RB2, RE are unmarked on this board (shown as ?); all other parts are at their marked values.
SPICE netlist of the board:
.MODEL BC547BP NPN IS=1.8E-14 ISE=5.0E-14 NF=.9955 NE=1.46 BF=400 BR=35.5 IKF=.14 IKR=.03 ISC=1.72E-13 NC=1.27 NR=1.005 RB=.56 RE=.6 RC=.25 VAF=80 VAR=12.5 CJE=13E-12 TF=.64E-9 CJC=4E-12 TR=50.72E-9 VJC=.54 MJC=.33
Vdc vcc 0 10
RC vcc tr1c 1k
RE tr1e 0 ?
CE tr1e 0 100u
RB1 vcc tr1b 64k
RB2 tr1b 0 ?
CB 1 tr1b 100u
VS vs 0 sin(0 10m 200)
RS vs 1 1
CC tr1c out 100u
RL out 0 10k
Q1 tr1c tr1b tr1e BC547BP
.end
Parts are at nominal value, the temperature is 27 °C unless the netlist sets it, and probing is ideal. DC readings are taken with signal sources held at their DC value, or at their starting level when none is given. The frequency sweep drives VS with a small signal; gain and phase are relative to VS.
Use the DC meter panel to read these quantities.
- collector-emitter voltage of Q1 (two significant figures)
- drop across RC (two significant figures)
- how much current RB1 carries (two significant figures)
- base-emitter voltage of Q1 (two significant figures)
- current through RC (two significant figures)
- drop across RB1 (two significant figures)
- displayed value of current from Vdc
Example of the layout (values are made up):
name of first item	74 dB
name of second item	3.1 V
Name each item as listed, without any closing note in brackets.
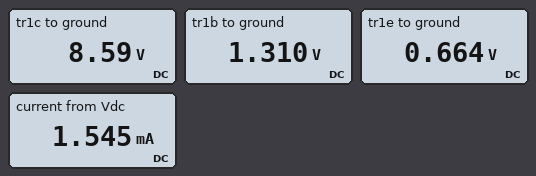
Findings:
collector-emitter voltage of Q1	7.9 V
drop across RC	1.4 V
how much current RB1 carries	140 µA
base-emitter voltage of Q1	650 mV
current through RC	1.4 mA
drop across RB1	8.7 V
displayed value of current from Vdc	1.545 mA
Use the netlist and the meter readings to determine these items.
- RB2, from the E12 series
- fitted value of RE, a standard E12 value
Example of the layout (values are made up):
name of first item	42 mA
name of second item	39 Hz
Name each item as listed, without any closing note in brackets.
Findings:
RB2, from the E12 series	10 kΩ
fitted value of RE, a standard E12 value	470 Ω
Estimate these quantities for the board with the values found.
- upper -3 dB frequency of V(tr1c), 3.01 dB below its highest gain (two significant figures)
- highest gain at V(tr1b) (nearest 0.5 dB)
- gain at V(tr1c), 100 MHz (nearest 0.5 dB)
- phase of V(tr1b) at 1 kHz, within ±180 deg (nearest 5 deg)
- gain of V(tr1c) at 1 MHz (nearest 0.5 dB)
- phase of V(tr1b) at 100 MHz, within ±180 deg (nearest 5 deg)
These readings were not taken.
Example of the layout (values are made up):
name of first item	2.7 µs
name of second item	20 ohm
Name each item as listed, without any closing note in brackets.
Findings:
upper -3 dB frequency of V(tr1c), 3.01 dB below its highest gain	98 MHz
highest gain at V(tr1b)	0 dB
gain at V(tr1c), 100 MHz	30.5 dB
phase of V(tr1b) at 1 kHz, within ±180 deg	0 deg
gain of V(tr1c) at 1 MHz	33.5 dB
phase of V(tr1b) at 100 MHz, within ±180 deg	-5 deg
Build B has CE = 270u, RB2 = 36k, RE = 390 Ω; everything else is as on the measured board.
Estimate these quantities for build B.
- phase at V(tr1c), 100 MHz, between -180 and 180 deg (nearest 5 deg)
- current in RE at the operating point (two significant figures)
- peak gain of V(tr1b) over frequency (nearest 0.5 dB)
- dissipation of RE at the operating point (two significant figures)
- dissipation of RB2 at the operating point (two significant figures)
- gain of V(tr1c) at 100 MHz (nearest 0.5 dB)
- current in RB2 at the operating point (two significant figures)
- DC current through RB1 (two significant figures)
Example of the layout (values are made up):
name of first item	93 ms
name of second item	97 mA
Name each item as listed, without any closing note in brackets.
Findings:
phase at V(tr1c), 100 MHz, between -180 and 180 deg	105 deg
current in RE at the operating point	6.2 mA
peak gain of V(tr1b) over frequency	0 dB
dissipation of RE at the operating point	15 mW
dissipation of RB2 at the operating point	270 µW
gain of V(tr1c) at 100 MHz	37.0 dB
current in RB2 at the operating point	87 µA
DC current through RB1	110 µA
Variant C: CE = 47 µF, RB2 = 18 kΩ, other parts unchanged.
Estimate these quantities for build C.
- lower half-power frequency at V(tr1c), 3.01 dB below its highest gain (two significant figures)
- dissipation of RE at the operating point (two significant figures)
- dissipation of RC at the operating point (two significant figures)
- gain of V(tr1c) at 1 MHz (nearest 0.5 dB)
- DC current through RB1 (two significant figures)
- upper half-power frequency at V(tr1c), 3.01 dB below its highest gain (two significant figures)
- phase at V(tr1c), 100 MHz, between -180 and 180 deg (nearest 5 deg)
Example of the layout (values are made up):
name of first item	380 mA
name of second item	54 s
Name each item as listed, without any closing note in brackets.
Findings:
lower half-power frequency at V(tr1c), 3.01 dB below its highest gain	350 Hz
dissipation of RE at the operating point	4.1 mW
dissipation of RC at the operating point	8.7 mW
gain of V(tr1c) at 1 MHz	39.5 dB
DC current through RB1	120 µA
upper half-power frequency at V(tr1c), 3.01 dB below its highest gain	82 MHz
phase at V(tr1c), 100 MHz, between -180 and 180 deg	125 deg
